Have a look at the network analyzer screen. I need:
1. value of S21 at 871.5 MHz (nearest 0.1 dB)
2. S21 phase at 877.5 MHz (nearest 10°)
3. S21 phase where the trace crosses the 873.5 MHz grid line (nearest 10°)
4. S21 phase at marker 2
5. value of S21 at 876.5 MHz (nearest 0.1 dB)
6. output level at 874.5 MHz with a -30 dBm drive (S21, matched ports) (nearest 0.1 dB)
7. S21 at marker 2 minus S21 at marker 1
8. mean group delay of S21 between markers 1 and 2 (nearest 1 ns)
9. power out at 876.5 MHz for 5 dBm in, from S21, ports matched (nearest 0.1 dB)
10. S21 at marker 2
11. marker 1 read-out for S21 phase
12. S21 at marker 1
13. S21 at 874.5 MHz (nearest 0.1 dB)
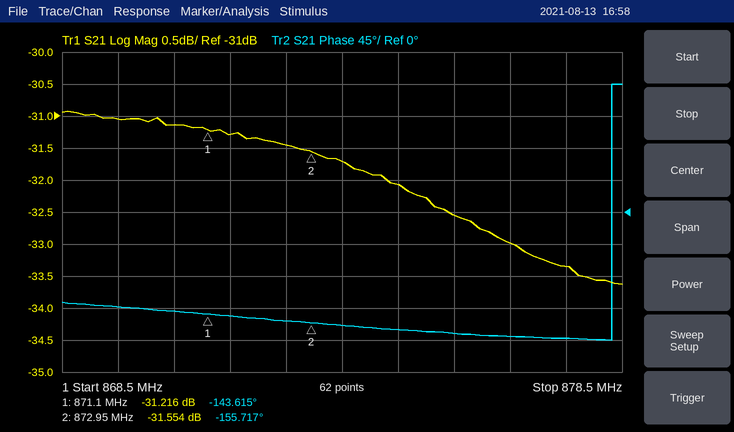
-31.3 dB
-180°
-160°
-155.717°
-33.0 dB
-62.1 dBm
-0.338 dB
18 ns
-28.0 dBm
-31.554 dB
-143.615°
-31.216 dB
-32.1 dB
